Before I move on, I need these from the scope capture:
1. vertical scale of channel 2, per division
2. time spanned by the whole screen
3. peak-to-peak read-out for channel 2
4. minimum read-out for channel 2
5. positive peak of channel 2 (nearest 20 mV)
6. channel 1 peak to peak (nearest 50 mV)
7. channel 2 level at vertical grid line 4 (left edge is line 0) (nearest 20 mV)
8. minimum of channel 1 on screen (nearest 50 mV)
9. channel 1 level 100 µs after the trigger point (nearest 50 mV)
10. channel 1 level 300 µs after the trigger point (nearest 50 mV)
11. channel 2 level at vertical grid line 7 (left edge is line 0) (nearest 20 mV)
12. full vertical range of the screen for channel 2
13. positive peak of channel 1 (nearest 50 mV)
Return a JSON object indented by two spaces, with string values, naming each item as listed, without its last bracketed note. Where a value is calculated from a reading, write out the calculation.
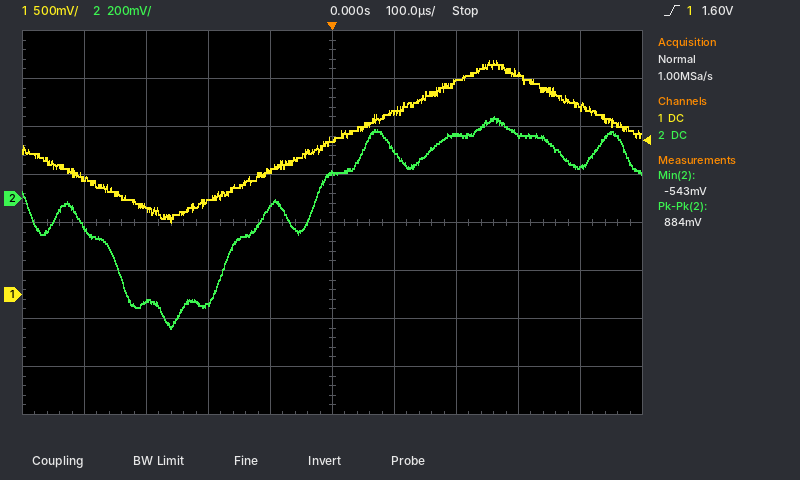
{
  "vertical scale of channel 2, per division": "200 mV",
  "time spanned by the whole screen": "1 ms",
  "peak-to-peak read-out for channel 2": "884 mV",
  "minimum read-out for channel 2": "-543 mV",
  "positive peak of channel 2": "340 mV",
  "channel 1 peak to peak": "2.45 V − (750 mV) = 1.70 V",
  "channel 2 level at vertical grid line 4 (left edge is line 0)": "-40 mV",
  "minimum of channel 1 on screen": "750 mV",
  "channel 1 level 100 µs after the trigger point": "1.90 V",
  "channel 1 level 300 µs after the trigger point": "2.30 V",
  "channel 2 level at vertical grid line 7 (left edge is line 0)": "260 mV",
  "full vertical range of the screen for channel 2": "1.6 V",
  "positive peak of channel 1": "2.45 V"
}
